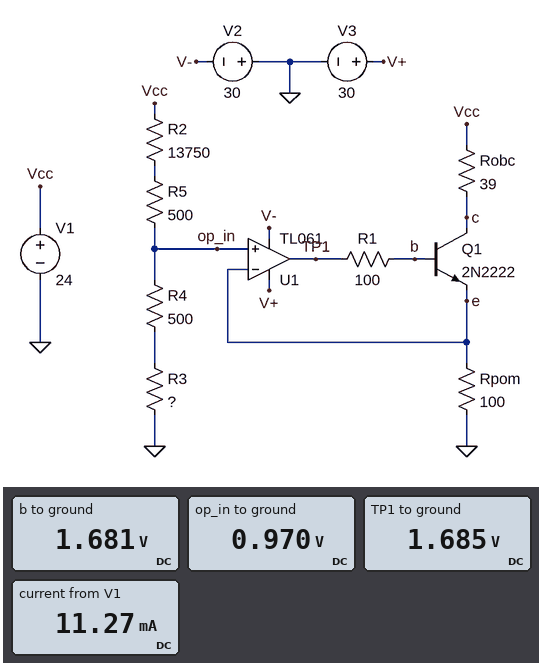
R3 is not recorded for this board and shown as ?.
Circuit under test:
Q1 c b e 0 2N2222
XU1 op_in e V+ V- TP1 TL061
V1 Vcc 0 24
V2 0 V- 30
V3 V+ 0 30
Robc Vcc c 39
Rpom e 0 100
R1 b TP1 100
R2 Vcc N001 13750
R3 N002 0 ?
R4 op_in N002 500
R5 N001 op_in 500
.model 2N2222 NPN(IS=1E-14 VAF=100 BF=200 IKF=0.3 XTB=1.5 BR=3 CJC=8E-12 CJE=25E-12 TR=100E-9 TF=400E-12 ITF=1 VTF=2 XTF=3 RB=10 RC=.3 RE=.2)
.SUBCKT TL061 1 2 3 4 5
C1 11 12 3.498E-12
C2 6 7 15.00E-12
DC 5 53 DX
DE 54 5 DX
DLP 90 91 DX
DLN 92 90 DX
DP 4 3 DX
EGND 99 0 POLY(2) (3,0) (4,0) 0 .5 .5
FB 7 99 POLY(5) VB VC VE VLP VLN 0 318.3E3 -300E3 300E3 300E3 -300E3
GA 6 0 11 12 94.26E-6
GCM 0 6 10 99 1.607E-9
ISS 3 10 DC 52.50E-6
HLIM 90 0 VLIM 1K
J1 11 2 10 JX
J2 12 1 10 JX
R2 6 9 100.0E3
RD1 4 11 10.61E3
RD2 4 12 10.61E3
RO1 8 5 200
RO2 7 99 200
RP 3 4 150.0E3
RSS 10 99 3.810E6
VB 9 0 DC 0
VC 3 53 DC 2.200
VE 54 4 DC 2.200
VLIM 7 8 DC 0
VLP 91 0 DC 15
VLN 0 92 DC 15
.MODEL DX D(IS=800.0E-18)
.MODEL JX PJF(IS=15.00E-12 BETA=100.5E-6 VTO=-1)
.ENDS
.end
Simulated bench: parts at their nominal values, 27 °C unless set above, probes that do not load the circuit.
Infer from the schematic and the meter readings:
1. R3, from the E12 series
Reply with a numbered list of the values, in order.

1. 100 Ω
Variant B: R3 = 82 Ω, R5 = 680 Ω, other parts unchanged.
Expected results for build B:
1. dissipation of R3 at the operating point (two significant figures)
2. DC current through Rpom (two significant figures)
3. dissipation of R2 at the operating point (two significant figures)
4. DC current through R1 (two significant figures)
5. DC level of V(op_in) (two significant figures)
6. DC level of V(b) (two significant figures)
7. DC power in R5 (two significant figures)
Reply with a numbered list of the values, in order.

1. 210 µW
2. 9.3 mA
3. 35 mW
4. 39 µA
5. 930 mV
6. 1.6 V
7. 1.7 mW
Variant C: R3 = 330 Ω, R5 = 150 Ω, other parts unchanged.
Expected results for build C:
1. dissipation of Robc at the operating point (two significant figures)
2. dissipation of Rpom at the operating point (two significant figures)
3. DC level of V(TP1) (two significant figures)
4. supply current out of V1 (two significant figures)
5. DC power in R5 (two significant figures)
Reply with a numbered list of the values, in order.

1. 7.1 mW
2. 18 mW
3. 2.1 V
4. 15 mA
5. 400 µW
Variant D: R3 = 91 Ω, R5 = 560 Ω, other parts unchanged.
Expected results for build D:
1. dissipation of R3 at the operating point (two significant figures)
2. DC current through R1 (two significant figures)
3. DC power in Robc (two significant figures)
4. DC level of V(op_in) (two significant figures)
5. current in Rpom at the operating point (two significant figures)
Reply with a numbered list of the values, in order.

1. 240 µW
2. 40 µA
3. 3.5 mW
4. 950 mV
5. 9.5 mA
